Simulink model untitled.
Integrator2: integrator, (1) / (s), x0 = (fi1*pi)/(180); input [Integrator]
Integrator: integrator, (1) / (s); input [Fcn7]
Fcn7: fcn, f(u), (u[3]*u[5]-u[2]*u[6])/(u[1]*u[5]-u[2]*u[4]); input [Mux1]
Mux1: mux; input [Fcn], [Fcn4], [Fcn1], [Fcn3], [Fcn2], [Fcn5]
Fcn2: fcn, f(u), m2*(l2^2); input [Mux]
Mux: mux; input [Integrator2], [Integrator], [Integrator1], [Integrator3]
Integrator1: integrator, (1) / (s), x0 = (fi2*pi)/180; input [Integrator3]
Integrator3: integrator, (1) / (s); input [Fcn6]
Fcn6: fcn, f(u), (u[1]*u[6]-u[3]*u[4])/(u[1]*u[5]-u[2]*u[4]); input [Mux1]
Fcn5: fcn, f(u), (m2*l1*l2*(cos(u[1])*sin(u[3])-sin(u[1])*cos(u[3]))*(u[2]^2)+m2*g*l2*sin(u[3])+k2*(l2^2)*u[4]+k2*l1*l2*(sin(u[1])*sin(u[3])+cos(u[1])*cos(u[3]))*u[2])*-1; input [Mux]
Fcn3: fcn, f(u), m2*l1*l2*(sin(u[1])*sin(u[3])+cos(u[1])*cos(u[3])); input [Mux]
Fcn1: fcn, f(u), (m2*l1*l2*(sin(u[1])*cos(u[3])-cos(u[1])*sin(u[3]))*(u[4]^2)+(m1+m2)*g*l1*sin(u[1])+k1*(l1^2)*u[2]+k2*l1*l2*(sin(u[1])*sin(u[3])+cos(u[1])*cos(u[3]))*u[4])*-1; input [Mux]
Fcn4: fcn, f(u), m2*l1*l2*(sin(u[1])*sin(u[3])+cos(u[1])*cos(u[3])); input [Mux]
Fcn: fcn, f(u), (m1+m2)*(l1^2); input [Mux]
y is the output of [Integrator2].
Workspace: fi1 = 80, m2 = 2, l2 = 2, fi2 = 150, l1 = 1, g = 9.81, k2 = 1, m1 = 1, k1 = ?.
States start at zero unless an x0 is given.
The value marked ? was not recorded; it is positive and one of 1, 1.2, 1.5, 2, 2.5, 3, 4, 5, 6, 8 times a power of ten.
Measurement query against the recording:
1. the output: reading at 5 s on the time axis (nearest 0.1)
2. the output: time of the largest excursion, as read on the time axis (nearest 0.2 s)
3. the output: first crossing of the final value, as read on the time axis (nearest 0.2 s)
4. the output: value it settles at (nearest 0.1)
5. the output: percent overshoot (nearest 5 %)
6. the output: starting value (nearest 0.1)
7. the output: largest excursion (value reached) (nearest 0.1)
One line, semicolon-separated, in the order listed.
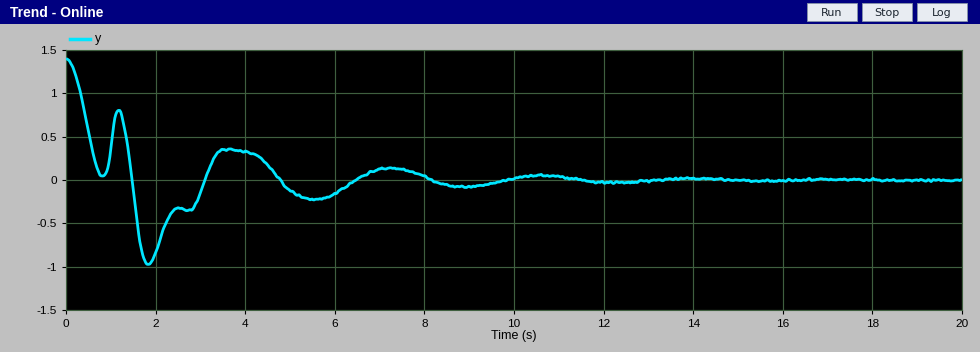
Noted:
-0.1; 1.8 s; 1.4 s; 0.0; 70 %; 1.4; -1.0
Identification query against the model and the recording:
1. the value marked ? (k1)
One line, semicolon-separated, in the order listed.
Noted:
4
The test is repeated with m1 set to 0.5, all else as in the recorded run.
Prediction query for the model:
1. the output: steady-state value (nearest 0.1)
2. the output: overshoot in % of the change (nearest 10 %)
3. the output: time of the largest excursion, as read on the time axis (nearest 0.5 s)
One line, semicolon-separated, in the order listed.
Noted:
0.0; 50 %; 2.5 s
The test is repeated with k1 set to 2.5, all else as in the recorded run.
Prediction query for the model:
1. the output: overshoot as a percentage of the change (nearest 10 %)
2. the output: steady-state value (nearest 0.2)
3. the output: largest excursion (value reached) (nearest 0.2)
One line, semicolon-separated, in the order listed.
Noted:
100 %; 0.0; -1.4
